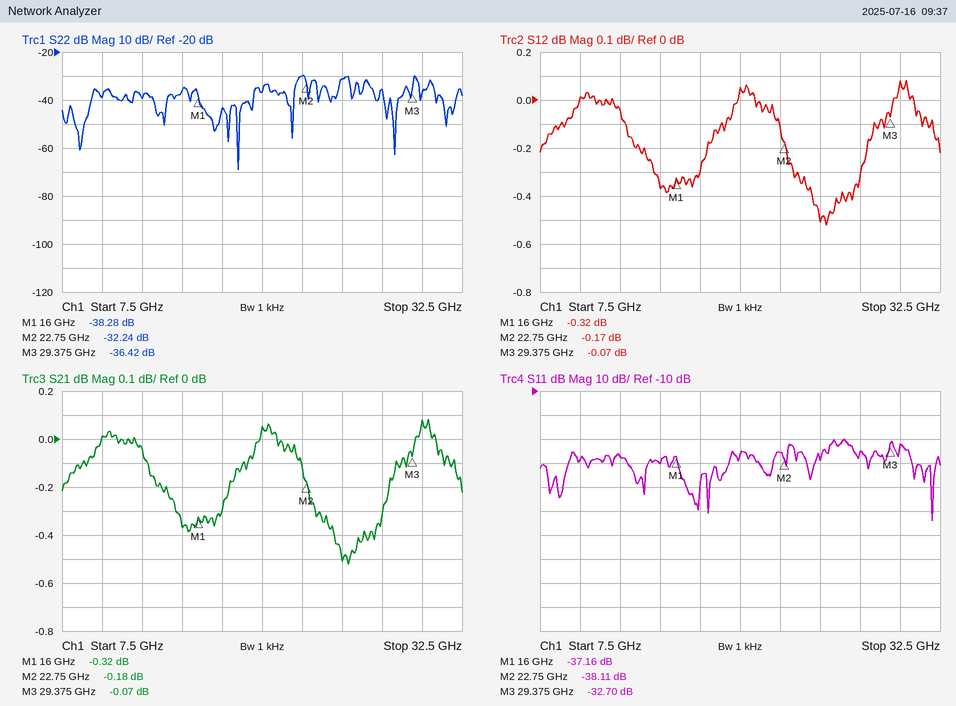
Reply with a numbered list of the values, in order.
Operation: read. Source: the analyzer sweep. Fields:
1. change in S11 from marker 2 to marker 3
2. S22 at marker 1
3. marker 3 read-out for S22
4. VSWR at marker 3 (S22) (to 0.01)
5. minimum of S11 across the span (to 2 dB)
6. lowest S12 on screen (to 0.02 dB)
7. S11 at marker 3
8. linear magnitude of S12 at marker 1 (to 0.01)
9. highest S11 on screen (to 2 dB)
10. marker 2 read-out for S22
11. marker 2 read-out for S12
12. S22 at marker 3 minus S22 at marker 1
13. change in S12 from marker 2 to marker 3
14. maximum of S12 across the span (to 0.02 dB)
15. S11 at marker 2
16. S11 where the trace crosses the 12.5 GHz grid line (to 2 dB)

1. 5.41 dB
2. -38.28 dB
3. -36.42 dB
4. 1.03
5. -64 dB
6. -0.52 dB
7. -32.70 dB
8. 0.96
9. -30 dB
10. -32.24 dB
11. -0.17 dB
12. 1.86 dB
13. 0.10 dB
14. 0.08 dB
15. -38.11 dB
16. -38 dB
